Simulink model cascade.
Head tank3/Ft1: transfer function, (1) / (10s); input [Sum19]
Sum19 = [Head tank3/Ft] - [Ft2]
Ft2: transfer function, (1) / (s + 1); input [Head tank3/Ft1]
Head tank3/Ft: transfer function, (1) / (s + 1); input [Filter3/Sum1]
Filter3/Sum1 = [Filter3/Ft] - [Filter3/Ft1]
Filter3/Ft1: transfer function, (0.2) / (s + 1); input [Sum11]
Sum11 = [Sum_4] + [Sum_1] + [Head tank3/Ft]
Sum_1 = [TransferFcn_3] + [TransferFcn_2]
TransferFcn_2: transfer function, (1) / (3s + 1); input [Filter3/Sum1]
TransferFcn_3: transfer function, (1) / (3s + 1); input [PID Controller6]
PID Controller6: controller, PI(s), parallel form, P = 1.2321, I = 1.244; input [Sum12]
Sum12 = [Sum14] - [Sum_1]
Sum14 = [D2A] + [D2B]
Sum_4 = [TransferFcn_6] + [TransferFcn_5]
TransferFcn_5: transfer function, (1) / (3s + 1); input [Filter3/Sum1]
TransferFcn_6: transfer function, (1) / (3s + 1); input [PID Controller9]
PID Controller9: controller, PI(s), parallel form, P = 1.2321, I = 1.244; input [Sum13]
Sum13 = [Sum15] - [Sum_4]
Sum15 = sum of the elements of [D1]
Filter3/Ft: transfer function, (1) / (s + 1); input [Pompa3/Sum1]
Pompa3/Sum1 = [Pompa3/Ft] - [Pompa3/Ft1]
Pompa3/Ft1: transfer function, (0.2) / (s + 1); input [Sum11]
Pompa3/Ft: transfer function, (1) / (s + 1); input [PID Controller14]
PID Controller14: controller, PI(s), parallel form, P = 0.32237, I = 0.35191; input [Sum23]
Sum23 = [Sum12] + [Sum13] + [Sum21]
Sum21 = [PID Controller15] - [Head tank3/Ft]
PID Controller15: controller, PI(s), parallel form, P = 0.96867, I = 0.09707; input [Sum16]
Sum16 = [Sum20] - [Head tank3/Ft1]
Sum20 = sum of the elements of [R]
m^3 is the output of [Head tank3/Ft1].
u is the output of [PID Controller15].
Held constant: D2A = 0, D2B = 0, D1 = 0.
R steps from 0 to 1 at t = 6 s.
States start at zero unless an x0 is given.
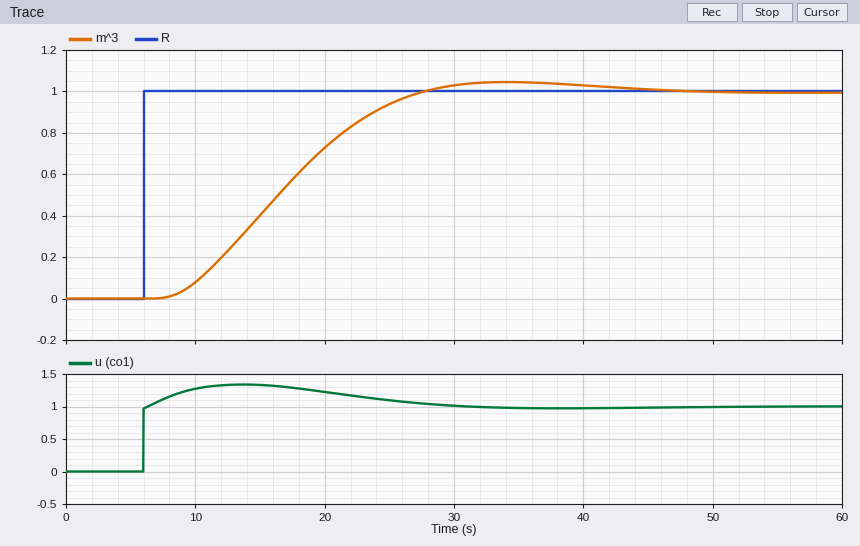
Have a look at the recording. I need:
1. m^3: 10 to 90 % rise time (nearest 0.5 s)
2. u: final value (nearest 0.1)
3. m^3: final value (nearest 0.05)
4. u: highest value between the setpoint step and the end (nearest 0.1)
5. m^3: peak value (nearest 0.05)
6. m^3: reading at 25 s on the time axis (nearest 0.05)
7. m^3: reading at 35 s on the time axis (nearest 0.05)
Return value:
13.5 s
1.0
1.00
1.3
1.05
0.95
1.05
